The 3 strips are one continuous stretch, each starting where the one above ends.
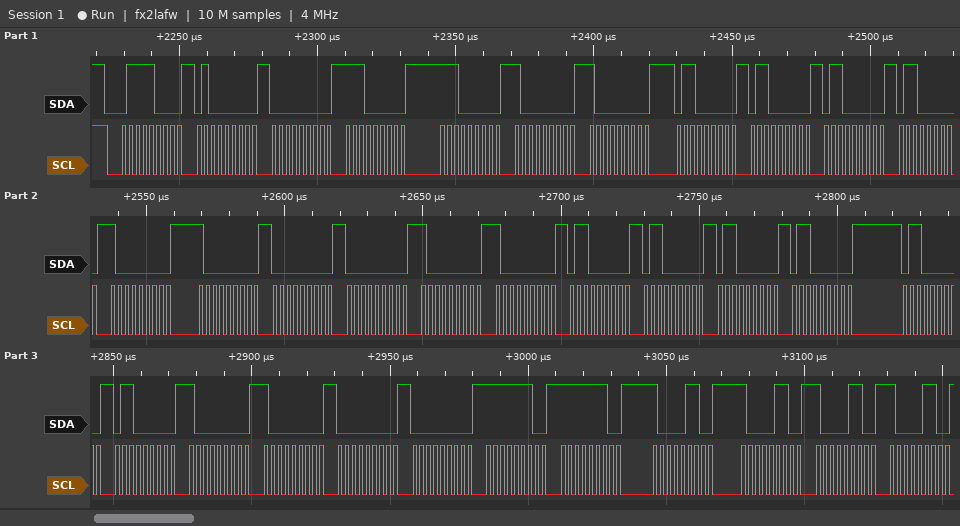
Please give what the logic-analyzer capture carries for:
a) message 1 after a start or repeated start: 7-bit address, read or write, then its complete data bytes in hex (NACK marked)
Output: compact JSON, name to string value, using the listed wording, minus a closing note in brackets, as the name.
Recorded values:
{"message 1 after a start or repeated start: 7-bit address, read or write, then its complete data bytes in hex": "0x3C write: 40 00 E0 E0 80 80 60 60 60 60 80 80 00 00 80 80 60 60 60 60 60 60 80 80 00 00 FE FE 86 86 86 86"}
